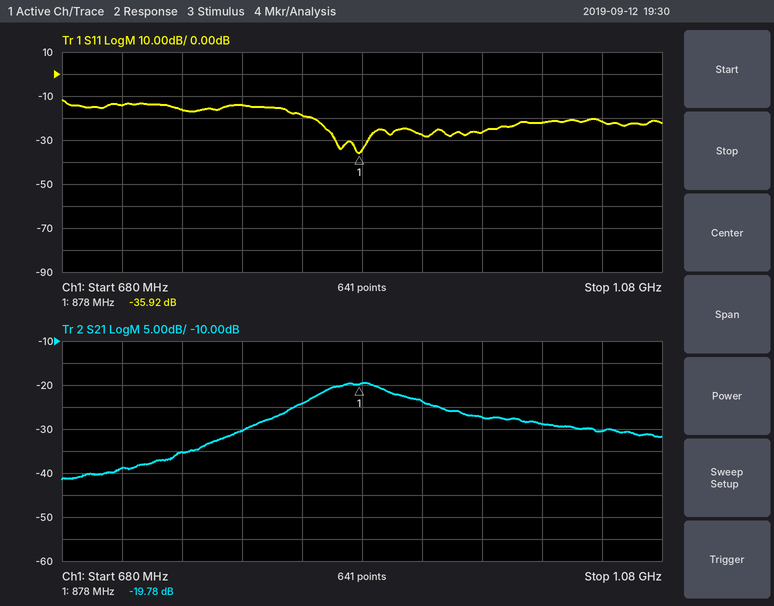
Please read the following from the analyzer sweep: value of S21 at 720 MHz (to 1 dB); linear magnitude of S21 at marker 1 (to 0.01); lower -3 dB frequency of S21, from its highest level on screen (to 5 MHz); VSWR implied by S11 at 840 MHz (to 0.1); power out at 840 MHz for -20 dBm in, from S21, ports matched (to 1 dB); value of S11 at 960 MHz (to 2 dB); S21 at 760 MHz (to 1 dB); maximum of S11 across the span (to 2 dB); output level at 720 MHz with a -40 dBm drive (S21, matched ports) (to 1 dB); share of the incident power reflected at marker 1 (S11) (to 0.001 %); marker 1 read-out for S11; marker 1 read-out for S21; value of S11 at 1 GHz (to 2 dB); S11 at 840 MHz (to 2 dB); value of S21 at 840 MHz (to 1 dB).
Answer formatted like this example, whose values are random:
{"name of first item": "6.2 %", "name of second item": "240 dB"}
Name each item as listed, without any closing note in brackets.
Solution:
{"value of S21 at 720 MHz": "-39 dB", "linear magnitude of S21 at marker 1": "0.10", "lower -3 dB frequency of S21, from its highest level on screen": "850 MHz", "VSWR implied by S11 at 840 MHz": "1.3", "power out at 840 MHz for -20 dBm in, from S21, ports matched": "-44 dBm", "value of S11 at 960 MHz": "-26 dB", "S21 at 760 MHz": "-35 dB", "maximum of S11 across the span": "-12 dB", "output level at 720 MHz with a -40 dBm drive (S21, matched ports)": "-79 dBm", "share of the incident power reflected at marker 1 (S11)": "0.026 %", "marker 1 read-out for S11": "-35.92 dB", "marker 1 read-out for S21": "-19.78 dB", "value of S11 at 1 GHz": "-22 dB", "S11 at 840 MHz": "-18 dB", "value of S21 at 840 MHz": "-24 dB"}
